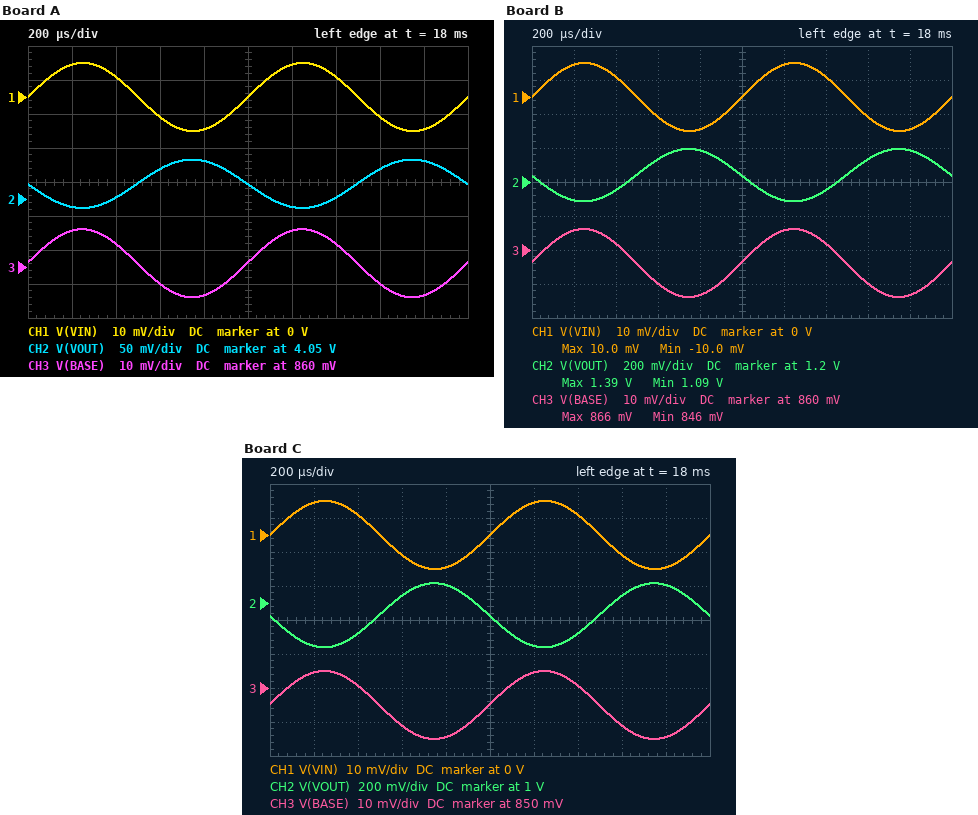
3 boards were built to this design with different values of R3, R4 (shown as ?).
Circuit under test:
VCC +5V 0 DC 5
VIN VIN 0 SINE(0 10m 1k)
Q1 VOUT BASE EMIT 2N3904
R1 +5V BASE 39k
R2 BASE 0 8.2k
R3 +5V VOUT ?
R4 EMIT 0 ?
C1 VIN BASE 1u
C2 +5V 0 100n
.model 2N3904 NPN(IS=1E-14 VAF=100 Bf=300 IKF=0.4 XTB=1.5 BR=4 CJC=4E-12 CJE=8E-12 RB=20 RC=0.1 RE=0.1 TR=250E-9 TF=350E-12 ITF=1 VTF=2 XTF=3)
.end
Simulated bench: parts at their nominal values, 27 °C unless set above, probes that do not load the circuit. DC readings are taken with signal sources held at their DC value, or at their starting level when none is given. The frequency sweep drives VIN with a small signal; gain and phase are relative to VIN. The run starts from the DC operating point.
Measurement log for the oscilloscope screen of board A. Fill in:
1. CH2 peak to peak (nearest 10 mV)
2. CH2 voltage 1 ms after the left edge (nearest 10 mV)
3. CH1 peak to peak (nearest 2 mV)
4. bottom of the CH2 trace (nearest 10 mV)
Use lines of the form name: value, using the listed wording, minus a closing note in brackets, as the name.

CH2 peak to peak: 70 mV
CH2 voltage 1 ms after the left edge: 4.07 V
CH1 peak to peak: 20 mV
bottom of the CH2 trace: 4.04 V
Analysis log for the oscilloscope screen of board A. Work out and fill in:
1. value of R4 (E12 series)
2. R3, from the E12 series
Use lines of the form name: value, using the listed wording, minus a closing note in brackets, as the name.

value of R4: 680 Ω
R3, from the E12 series: 2.7 kΩ
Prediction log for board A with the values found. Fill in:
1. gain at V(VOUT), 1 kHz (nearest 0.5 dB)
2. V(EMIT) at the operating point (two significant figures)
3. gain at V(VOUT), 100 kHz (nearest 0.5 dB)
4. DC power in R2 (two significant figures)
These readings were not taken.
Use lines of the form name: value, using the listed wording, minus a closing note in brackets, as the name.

gain at V(VOUT), 1 kHz: 11.0 dB
V(EMIT) at the operating point: 230 mV
gain at V(VOUT), 100 kHz: 11.0 dB
DC power in R2: 90 µW
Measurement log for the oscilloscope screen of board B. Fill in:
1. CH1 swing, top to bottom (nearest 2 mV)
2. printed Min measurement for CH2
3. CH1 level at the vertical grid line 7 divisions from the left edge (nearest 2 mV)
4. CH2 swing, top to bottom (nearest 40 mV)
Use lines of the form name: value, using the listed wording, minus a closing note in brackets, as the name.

CH1 swing, top to bottom: 20 mV
printed Min measurement for CH2: 1.09 V
CH1 level at the vertical grid line 7 divisions from the left edge: 6 mV
CH2 swing, top to bottom: 320 mV
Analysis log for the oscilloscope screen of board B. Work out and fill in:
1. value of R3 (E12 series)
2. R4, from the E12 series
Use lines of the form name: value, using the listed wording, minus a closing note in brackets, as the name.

value of R3: 6.8 kΩ
R4, from the E12 series: 390 Ω
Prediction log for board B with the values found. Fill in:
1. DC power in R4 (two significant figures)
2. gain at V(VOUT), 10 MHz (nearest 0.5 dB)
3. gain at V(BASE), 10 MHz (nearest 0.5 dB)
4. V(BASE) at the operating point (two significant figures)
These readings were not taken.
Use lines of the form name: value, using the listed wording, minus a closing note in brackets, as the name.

DC power in R4: 120 µW
gain at V(VOUT), 10 MHz: 18.5 dB
gain at V(BASE), 10 MHz: 0 dB
V(BASE) at the operating point: 860 mV
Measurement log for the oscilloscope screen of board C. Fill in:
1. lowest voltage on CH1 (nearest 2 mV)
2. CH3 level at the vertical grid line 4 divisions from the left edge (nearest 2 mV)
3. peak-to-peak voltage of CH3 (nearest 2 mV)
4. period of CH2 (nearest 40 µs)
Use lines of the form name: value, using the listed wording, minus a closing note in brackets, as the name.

lowest voltage on CH1: -10 mV
CH3 level at the vertical grid line 4 divisions from the left edge: 836 mV
peak-to-peak voltage of CH3: 20 mV
period of CH2: 1.00 ms
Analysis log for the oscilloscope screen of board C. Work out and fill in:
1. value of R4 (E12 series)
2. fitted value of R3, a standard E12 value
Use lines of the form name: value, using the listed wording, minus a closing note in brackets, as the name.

value of R4: 180 Ω
fitted value of R3, a standard E12 value: 3.9 kΩ
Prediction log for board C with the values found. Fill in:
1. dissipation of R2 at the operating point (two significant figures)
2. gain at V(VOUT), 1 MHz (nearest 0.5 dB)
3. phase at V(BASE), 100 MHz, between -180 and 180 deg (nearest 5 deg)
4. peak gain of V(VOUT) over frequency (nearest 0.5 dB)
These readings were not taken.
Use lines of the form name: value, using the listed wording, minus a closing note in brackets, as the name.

dissipation of R2 at the operating point: 87 µW
gain at V(VOUT), 1 MHz: 25.5 dB
phase at V(BASE), 100 MHz, between -180 and 180 deg: 0 deg
peak gain of V(VOUT) over frequency: 25.5 dB
